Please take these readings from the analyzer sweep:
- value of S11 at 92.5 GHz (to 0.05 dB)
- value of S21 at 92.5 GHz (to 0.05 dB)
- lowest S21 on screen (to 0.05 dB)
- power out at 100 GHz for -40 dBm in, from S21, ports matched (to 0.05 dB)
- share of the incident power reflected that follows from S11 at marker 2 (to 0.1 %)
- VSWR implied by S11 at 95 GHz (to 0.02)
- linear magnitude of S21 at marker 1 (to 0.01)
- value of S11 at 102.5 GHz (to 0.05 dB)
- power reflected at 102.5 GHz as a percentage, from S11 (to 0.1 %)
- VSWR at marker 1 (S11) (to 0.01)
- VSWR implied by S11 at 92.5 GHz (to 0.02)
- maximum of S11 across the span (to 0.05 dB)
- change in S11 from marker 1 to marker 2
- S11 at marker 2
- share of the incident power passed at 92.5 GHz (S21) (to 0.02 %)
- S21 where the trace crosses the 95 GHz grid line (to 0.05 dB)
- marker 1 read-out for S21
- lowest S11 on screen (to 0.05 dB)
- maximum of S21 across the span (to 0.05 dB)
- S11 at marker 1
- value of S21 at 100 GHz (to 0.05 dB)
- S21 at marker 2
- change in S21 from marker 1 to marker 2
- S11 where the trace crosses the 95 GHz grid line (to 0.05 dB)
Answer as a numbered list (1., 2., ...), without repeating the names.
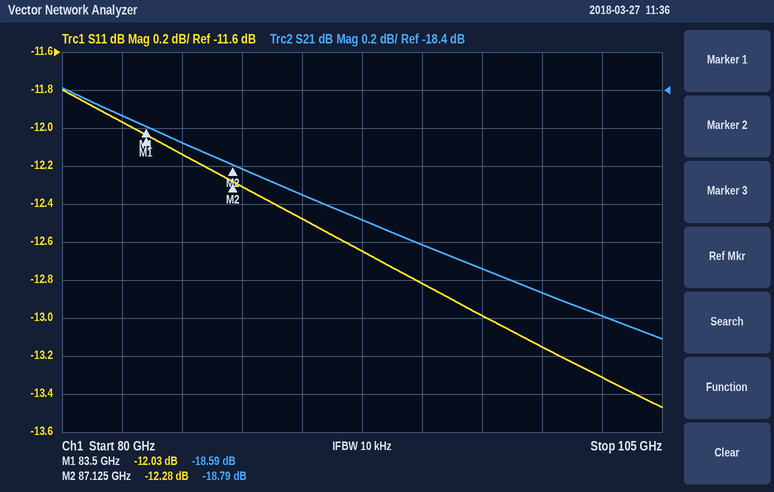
1. -12.65 dB
2. -19.10 dB
3. -19.70 dB
4. -59.45 dBm
5. 5.9 %
6. 1.60
7. 0.12
8. -13.30 dB
9. 4.7 %
10. 1.67
11. 1.60
12. -11.80 dB
13. -0.25 dB
14. -12.28 dB
15. 1.24 %
16. -19.20 dB
17. -18.59 dB
18. -13.45 dB
19. -18.40 dB
20. -12.03 dB
21. -19.45 dB
22. -18.79 dB
23. -0.20 dB
24. -12.80 dB
